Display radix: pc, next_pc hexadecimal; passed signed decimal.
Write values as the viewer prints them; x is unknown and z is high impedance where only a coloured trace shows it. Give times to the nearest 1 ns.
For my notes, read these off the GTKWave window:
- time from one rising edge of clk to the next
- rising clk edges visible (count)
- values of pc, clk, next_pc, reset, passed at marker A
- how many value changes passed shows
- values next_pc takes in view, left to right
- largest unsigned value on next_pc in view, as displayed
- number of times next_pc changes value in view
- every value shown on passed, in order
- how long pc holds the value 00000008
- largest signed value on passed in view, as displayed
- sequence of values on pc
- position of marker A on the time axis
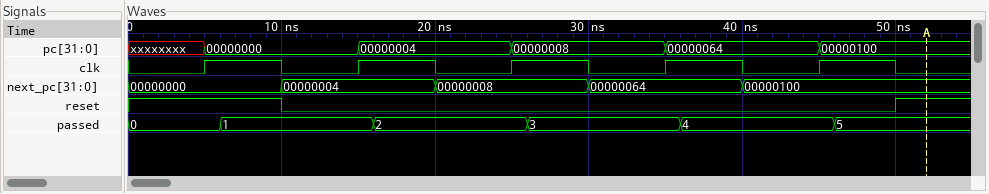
10 ns
5
pc=00000100, clk=0, next_pc=00000100, reset=1, passed=5
5
00000000, 00000004, 00000008, 00000064, 00000100
00000100
4
0, 1, 2, 3, 4, 5
10 ns
5
xxxxxxxx, 00000000, 00000004, 00000008, 00000064, 00000100
52 ns
